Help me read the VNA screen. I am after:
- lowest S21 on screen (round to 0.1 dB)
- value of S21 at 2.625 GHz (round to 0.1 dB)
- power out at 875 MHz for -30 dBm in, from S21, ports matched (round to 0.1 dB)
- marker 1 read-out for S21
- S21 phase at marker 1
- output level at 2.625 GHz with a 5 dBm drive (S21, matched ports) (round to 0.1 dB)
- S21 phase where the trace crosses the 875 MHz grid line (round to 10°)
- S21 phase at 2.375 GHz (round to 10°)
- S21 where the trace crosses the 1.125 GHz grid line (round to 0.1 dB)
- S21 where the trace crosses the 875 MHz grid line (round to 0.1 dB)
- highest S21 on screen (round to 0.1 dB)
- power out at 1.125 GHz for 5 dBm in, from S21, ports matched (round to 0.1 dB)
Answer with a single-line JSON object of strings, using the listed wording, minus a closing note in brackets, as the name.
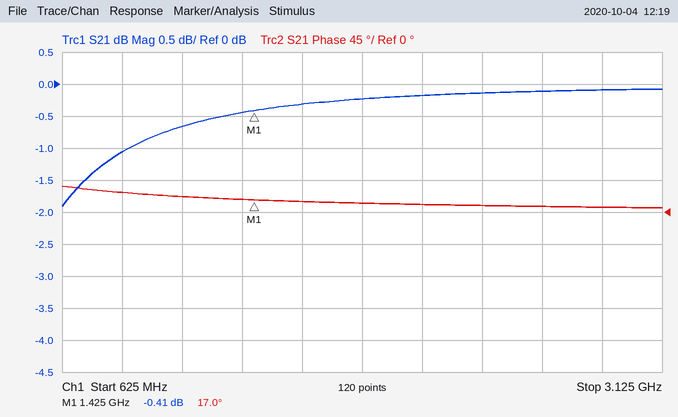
{"lowest S21 on screen": "-1.9 dB", "value of S21 at 2.625 GHz": "-0.1 dB", "power out at 875 MHz for -30 dBm in, from S21, ports matched": "-31.1 dBm", "marker 1 read-out for S21": "-0.41 dB", "S21 phase at marker 1": "17.0°", "output level at 2.625 GHz with a 5 dBm drive (S21, matched ports)": "4.9 dBm", "S21 phase where the trace crosses the 875 MHz grid line": "30°", "S21 phase at 2.375 GHz": "10°", "S21 where the trace crosses the 1.125 GHz grid line": "-0.7 dB", "S21 where the trace crosses the 875 MHz grid line": "-1.1 dB", "highest S21 on screen": "-0.1 dB", "power out at 1.125 GHz for 5 dBm in, from S21, ports matched": "4.3 dBm"}
